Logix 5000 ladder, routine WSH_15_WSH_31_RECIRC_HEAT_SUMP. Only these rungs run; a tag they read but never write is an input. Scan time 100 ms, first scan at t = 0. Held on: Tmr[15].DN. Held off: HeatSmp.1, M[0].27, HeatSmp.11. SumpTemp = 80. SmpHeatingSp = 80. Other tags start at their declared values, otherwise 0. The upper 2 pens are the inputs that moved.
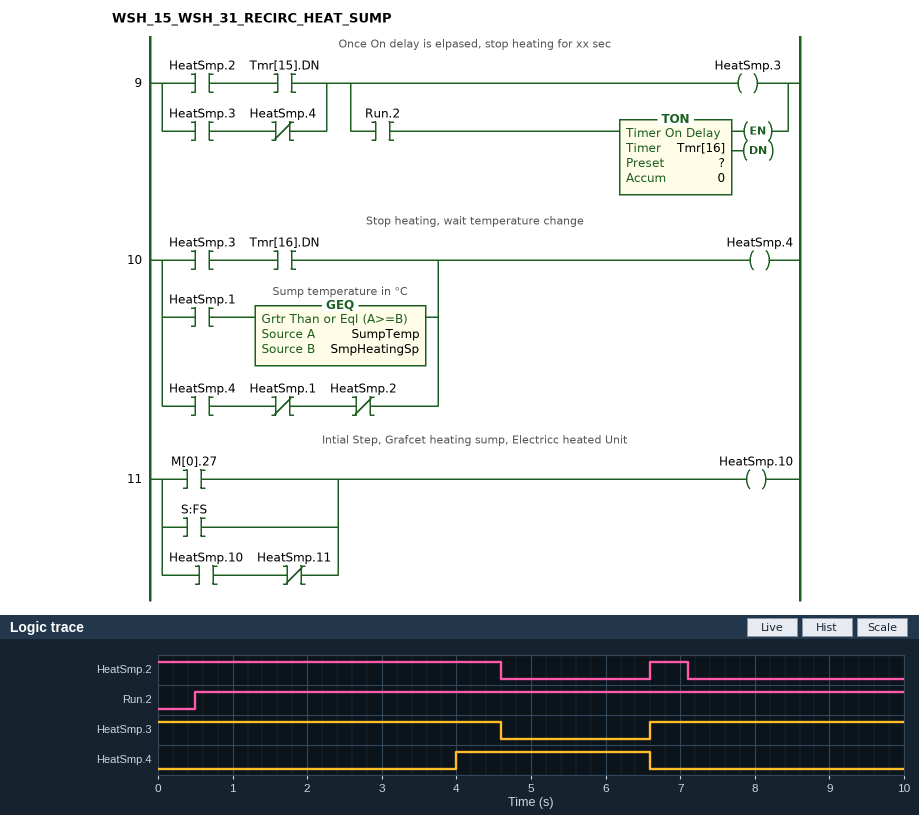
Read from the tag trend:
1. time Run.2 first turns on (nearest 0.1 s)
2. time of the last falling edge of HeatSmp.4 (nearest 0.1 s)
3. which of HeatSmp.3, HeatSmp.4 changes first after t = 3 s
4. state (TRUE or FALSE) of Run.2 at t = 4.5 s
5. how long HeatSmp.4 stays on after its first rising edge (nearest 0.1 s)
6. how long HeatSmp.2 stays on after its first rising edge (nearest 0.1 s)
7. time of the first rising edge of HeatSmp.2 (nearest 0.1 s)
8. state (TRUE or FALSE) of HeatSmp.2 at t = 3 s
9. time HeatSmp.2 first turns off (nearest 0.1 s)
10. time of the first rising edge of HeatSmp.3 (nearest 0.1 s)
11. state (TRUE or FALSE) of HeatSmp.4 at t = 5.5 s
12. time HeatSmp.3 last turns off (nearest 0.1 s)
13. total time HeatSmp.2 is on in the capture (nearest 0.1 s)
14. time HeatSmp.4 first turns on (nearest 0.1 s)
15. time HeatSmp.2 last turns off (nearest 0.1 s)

0.5 s
6.6 s
HeatSmp.4
TRUE
2.6 s
0.5 s
6.6 s
TRUE
4.6 s
6.6 s
TRUE
4.6 s
5.1 s
4.0 s
7.1 s
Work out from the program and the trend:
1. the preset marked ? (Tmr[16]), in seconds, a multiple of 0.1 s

3.5 s
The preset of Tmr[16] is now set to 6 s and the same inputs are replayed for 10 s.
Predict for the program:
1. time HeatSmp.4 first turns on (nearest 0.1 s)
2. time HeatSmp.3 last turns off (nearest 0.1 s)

6.5 s
7.1 s
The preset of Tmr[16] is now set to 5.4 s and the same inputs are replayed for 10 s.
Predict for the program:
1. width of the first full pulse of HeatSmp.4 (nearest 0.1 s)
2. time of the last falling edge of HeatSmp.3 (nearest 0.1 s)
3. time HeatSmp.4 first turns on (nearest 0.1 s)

0.7 s
6.0 s
5.9 s
